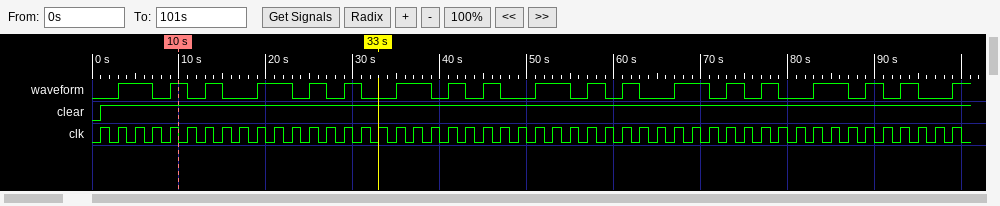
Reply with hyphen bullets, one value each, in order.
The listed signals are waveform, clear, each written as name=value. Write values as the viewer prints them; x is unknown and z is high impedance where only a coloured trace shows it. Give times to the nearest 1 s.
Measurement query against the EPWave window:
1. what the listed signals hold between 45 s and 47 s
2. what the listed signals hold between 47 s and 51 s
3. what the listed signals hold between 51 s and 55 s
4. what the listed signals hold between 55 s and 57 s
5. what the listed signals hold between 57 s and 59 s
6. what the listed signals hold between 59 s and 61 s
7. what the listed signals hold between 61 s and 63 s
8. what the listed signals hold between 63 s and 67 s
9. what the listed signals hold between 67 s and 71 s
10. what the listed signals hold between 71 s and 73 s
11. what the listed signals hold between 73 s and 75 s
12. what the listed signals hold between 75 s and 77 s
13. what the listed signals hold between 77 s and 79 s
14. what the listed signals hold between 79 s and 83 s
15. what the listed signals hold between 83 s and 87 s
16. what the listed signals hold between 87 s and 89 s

- waveform=1, clear=1
- waveform=0, clear=1
- waveform=1, clear=1
- waveform=0, clear=1
- waveform=1, clear=1
- waveform=0, clear=1
- waveform=1, clear=1
- waveform=0, clear=1
- waveform=1, clear=1
- waveform=0, clear=1
- waveform=1, clear=1
- waveform=0, clear=1
- waveform=1, clear=1
- waveform=0, clear=1
- waveform=1, clear=1
- waveform=0, clear=1
